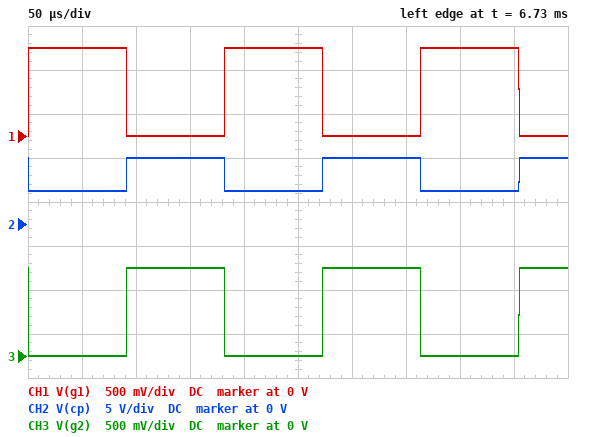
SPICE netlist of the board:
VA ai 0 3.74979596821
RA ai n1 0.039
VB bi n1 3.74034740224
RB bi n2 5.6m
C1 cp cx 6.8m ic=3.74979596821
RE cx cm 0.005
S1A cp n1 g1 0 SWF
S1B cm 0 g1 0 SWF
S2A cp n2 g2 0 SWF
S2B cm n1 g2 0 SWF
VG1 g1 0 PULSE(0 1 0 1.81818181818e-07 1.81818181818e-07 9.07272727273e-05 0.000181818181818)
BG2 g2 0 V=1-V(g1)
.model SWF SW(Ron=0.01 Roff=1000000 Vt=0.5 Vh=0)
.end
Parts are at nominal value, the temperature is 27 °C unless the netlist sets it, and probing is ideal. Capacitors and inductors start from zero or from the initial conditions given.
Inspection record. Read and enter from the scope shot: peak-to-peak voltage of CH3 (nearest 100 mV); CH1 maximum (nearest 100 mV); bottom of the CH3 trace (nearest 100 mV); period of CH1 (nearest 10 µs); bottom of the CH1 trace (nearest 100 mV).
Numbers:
1.0 V
1.0 V
0 V
180 µs
0 V
